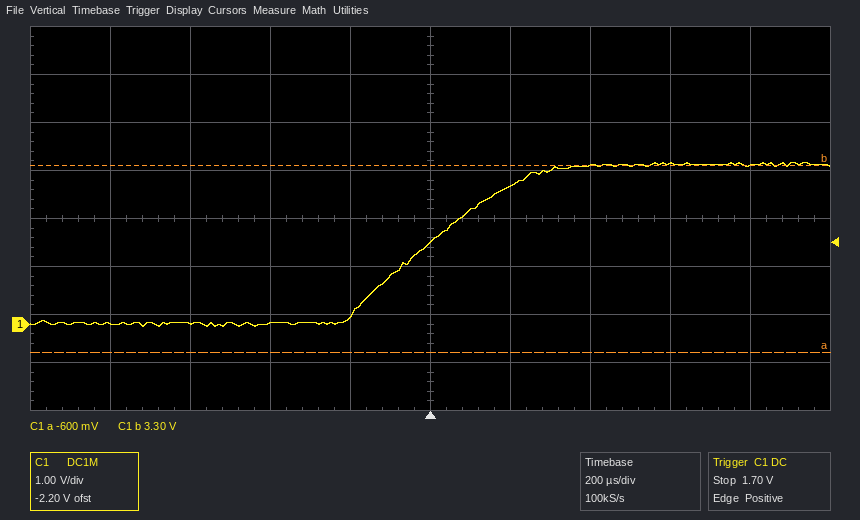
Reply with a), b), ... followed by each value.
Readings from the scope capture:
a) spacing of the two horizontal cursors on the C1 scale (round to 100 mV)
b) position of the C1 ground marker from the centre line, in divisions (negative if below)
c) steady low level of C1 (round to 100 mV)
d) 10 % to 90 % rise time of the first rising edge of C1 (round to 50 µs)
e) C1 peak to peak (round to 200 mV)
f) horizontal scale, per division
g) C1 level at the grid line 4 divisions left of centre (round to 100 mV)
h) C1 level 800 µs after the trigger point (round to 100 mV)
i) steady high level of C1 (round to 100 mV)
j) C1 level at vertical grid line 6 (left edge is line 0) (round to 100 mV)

a) 3.9 V
b) -2.2 div
c) 0.0 V
d) 400 µs
e) 3.4 V
f) 200 µs
g) 0.0 V
h) 3.3 V
i) 3.3 V
j) 2.9 V
